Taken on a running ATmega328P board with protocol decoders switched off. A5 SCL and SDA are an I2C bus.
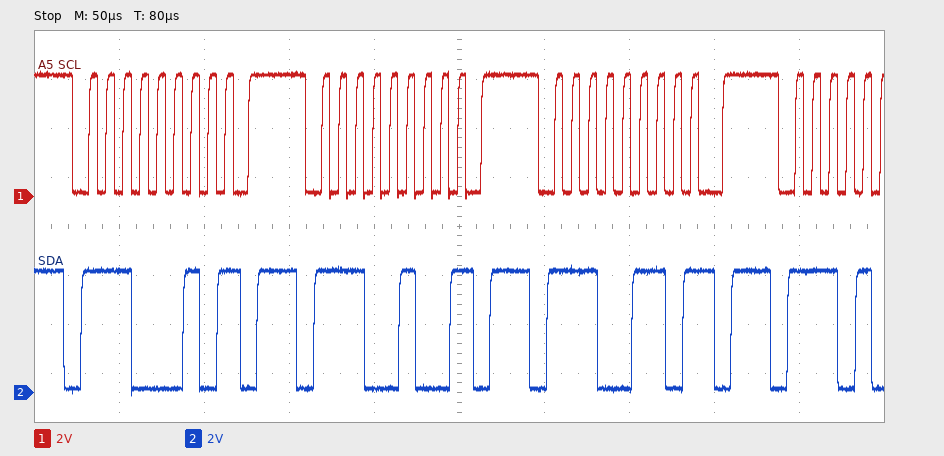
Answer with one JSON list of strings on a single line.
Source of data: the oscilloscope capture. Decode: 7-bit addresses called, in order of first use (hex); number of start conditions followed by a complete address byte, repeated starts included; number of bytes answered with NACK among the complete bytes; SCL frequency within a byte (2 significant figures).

["0x71 0x72 0x73", "3", "3", "100 kHz"]
